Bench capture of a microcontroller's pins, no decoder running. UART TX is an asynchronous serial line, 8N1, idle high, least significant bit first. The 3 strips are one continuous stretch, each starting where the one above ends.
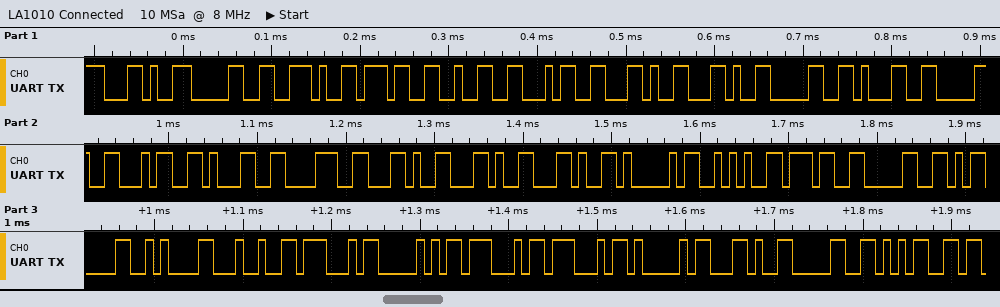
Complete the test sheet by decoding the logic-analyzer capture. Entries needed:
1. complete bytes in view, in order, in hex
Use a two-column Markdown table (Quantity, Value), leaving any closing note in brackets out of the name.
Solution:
| Quantity | Value |
|---|---|
| complete bytes in view, in order, in hex | 2C 30 2E 37 32 34 2C 2C 30 31 30 34 31 38 2C 2C 2C 41 2A 37 30 0D 0A 24 47 50 47 47 41 2C 30 35 |
